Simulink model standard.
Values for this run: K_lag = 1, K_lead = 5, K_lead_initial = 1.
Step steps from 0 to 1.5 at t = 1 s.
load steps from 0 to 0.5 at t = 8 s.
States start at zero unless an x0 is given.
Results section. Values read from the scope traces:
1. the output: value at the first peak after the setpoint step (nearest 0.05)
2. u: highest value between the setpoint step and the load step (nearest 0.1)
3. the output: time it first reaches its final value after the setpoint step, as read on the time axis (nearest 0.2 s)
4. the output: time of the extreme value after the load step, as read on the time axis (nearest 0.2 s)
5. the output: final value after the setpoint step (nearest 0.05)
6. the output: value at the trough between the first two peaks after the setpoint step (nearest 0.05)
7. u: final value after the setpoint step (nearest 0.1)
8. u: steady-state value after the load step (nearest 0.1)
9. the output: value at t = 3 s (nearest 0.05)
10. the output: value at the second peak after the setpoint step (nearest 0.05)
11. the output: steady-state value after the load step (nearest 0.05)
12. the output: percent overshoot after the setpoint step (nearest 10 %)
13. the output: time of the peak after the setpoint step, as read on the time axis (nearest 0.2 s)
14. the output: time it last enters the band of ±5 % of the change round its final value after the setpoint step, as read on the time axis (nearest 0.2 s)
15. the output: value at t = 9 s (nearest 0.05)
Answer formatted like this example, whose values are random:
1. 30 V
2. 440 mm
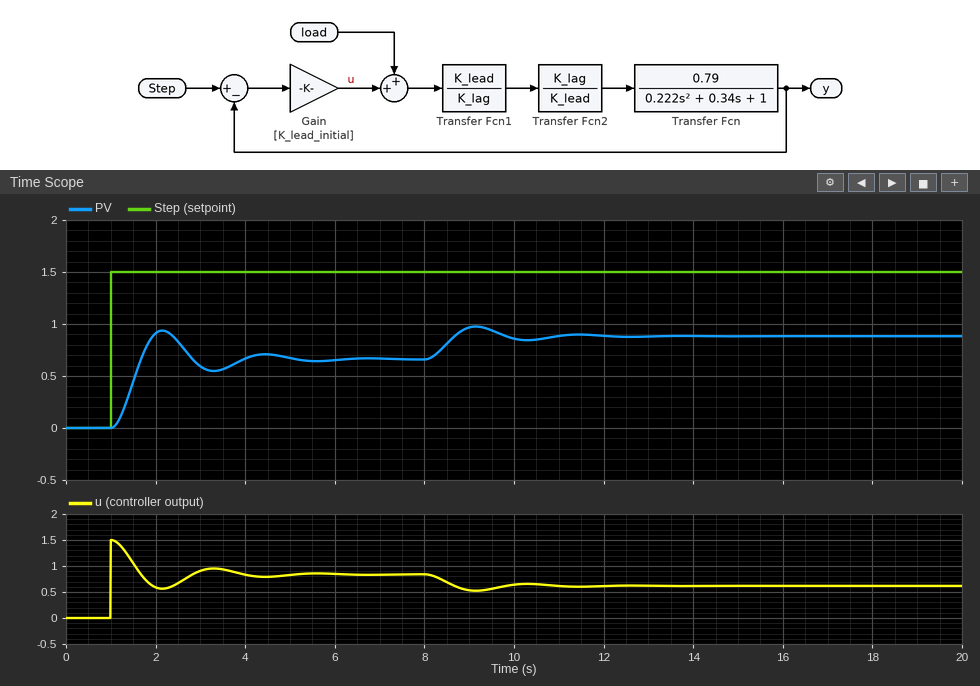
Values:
1. 0.95
2. 1.5
3. 1.6 s
4. 9.2 s
5. 0.65
6. 0.55
7. 0.8
8. 0.6
9. 0.60
10. 0.70
11. 0.90
12. 40 %
13. 2.2 s
14. 4.8 s
15. 0.95
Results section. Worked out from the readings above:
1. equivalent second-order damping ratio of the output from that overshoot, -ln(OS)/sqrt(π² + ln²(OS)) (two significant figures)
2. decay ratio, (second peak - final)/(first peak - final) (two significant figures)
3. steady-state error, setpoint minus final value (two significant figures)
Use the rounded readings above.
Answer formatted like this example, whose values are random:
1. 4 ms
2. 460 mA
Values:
1. 0.28
2. 0.17
3. 0.85
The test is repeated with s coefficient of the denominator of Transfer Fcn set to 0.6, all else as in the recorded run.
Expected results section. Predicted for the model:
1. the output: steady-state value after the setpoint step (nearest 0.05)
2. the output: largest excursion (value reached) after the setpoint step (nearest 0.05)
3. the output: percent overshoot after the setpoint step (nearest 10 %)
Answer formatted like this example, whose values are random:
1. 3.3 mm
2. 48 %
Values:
1. 0.65
2. 0.80
3. 20 %
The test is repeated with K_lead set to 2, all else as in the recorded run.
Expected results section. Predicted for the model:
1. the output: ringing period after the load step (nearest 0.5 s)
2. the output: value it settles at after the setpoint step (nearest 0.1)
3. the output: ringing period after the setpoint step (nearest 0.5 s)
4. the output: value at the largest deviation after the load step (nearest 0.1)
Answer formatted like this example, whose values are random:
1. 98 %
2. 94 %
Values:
1. 2.5 s
2. 0.7
3. 2.5 s
4. 1.0
